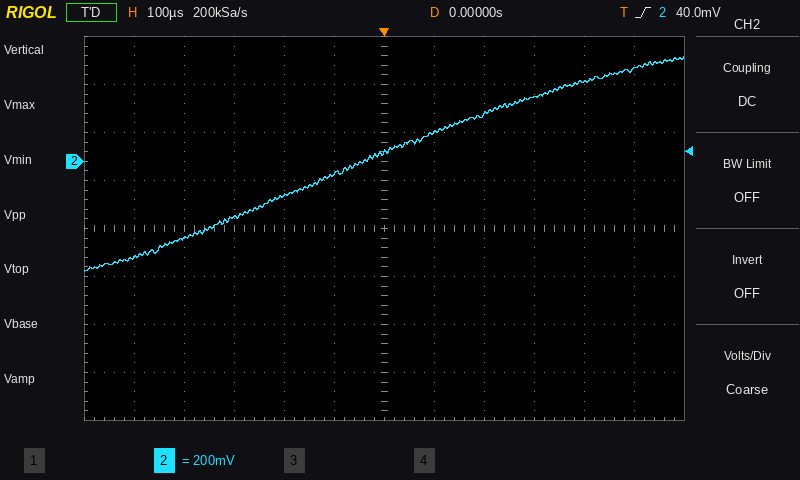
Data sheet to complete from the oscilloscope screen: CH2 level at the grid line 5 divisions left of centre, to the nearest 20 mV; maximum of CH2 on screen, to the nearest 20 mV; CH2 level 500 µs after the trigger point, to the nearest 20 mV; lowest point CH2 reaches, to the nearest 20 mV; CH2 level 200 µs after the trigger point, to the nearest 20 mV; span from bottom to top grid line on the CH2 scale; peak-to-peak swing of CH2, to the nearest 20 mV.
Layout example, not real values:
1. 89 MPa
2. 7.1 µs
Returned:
1. -400 mV
2. 440 mV
3. 380 mV
4. -460 mV
5. 200 mV
6. 1.6 V
7. 900 mV
